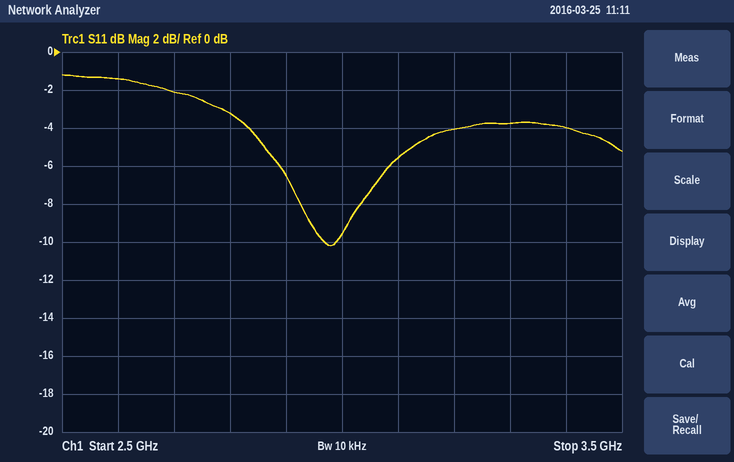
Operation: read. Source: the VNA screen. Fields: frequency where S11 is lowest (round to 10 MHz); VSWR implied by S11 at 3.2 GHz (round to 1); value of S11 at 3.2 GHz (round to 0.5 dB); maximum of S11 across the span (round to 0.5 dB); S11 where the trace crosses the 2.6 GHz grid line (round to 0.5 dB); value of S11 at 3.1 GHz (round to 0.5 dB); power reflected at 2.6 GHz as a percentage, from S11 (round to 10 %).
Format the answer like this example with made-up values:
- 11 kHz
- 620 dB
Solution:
- 2.98 GHz
- 4
- -4.0 dB
- -1.0 dB
- -1.5 dB
- -5.5 dB
- 70 %
